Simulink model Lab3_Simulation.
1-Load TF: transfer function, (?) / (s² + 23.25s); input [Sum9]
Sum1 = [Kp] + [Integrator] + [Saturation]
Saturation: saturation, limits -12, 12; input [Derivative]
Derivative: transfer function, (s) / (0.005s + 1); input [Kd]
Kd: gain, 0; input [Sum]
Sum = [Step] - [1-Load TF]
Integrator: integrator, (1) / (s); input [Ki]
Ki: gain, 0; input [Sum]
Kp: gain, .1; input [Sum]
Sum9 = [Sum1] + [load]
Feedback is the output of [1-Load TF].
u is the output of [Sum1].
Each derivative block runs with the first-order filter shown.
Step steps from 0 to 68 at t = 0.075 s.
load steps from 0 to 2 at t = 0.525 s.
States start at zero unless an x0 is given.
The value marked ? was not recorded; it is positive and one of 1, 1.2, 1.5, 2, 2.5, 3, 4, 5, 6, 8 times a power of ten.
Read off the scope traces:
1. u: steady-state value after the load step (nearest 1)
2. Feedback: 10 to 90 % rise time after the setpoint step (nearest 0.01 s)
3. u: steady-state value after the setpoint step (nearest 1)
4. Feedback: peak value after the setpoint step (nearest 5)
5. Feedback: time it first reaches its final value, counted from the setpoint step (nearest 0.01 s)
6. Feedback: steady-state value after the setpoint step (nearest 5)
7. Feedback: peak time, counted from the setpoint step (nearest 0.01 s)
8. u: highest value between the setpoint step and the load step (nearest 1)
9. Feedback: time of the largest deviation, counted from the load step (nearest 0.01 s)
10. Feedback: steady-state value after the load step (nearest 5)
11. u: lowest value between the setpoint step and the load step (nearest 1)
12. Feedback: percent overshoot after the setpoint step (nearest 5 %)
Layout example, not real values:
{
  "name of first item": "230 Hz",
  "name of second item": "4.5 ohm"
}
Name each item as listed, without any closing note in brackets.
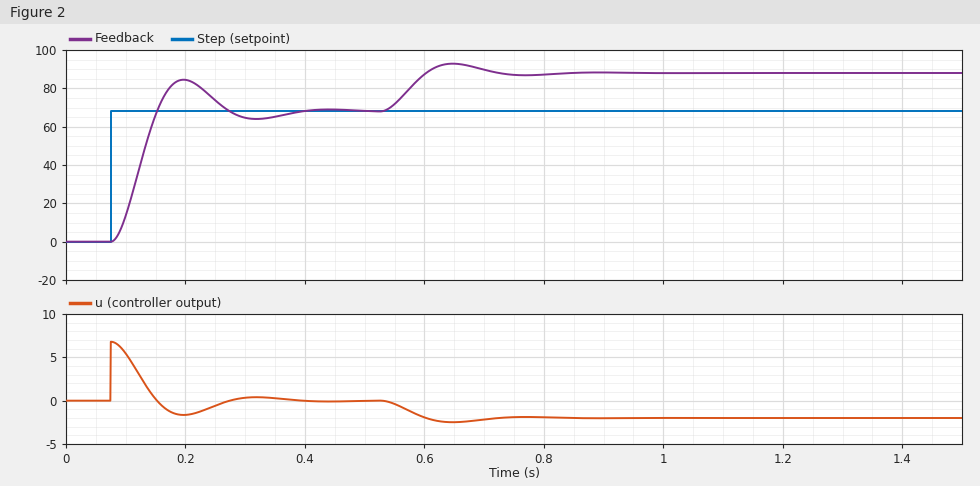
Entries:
{
  "u: steady-state value after the load step": "-2",
  "Feedback: 10 to 90 % rise time after the setpoint step": "0.05 s",
  "u: steady-state value after the setpoint step": "0",
  "Feedback: peak value after the setpoint step": "85",
  "Feedback: time it first reaches its final value, counted from the setpoint step": "0.08 s",
  "Feedback: steady-state value after the setpoint step": "70",
  "Feedback: peak time, counted from the setpoint step": "0.12 s",
  "u: highest value between the setpoint step and the load step": "7",
  "Feedback: time of the largest deviation, counted from the load step": "0.12 s",
  "Feedback: steady-state value after the load step": "90",
  "u: lowest value between the setpoint step and the load step": "-2",
  "Feedback: percent overshoot after the setpoint step": "25 %"
}
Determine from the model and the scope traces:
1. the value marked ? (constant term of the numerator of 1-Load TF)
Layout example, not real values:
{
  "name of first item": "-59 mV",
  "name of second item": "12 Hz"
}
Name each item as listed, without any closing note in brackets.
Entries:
{
  "the value marked ?": "8000"
}
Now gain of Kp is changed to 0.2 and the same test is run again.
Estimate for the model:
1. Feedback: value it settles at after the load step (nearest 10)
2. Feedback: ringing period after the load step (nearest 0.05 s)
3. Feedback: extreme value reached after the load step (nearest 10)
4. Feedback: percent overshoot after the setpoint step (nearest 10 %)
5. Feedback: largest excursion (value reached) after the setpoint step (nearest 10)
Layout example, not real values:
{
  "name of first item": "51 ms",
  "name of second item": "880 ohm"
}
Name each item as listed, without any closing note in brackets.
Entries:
{
  "Feedback: value it settles at after the load step": "80",
  "Feedback: ringing period after the load step": "0.15 s",
  "Feedback: extreme value reached after the load step": "80",
  "Feedback: percent overshoot after the setpoint step": "40 %",
  "Feedback: largest excursion (value reached) after the setpoint step": "90"
}
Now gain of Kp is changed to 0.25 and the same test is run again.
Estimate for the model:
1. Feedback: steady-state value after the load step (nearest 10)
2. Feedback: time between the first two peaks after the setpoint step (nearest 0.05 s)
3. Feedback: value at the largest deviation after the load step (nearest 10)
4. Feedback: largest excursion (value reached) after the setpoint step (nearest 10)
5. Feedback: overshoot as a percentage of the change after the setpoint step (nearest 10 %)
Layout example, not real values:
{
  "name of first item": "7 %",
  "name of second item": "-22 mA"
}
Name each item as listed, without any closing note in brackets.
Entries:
{
  "Feedback: steady-state value after the load step": "80",
  "Feedback: time between the first two peaks after the setpoint step": "0.15 s",
  "Feedback: value at the largest deviation after the load step": "80",
  "Feedback: largest excursion (value reached) after the setpoint step": "100",
  "Feedback: overshoot as a percentage of the change after the setpoint step": "40 %"
}
